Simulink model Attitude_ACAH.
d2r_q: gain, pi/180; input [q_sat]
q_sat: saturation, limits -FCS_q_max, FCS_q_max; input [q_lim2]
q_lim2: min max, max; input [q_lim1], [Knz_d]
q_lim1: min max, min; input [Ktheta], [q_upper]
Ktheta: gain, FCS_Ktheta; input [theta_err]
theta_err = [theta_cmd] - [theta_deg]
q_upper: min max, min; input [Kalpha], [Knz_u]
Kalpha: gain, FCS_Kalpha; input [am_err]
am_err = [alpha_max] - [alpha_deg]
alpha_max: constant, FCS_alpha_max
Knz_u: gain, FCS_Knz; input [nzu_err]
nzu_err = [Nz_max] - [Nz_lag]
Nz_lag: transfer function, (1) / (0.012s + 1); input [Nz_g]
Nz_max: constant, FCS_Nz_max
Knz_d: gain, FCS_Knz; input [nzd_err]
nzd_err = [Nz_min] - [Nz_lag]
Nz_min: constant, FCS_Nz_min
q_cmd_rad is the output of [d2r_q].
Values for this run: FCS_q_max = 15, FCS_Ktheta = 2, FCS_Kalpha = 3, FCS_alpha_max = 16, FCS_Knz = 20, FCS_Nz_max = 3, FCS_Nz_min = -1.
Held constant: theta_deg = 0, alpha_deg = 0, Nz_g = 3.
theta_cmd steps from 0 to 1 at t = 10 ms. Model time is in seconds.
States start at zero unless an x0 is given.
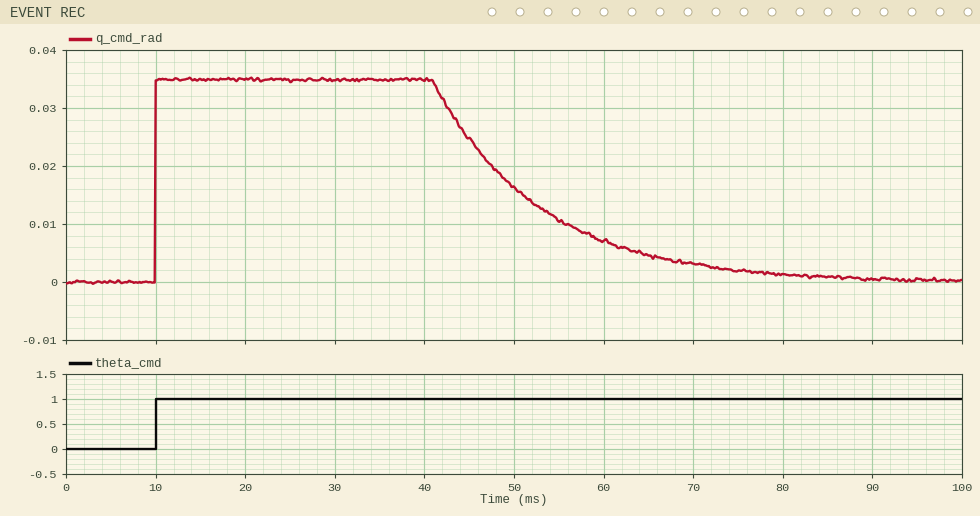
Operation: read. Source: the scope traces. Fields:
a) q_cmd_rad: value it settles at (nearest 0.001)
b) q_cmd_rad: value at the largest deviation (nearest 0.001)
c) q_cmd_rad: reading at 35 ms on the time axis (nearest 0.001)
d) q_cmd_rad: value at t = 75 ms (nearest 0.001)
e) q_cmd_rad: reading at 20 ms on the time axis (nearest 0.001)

0.000
0.035
0.035
0.002
0.035
